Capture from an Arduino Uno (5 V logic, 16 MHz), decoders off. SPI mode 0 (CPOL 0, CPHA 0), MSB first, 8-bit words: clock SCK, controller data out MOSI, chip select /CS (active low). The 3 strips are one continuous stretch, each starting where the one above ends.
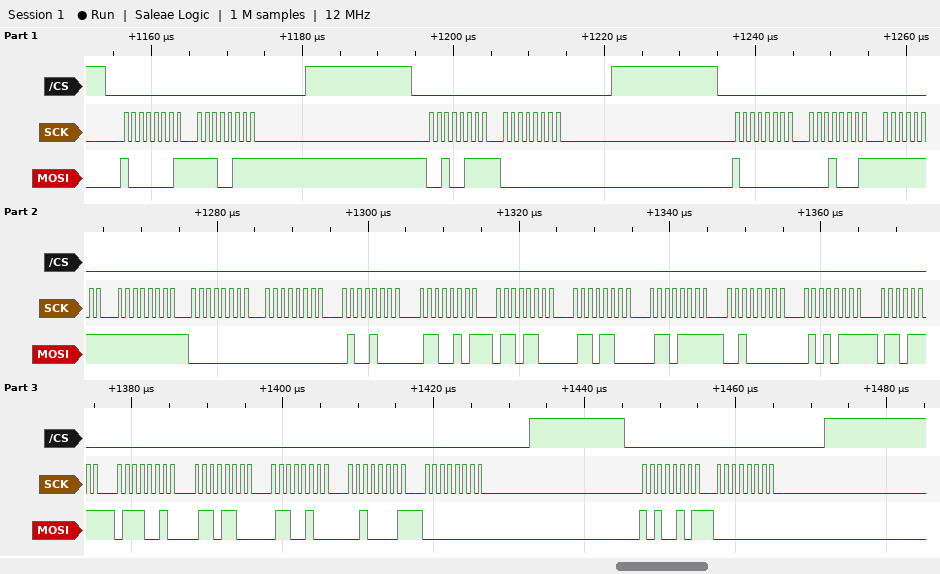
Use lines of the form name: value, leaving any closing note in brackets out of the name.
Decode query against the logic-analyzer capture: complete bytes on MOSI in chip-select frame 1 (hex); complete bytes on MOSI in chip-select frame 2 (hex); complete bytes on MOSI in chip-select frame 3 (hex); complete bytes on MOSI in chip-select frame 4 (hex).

complete bytes on MOSI in chip-select frame 1: 0x81 0xE7
complete bytes on MOSI in chip-select frame 2: 0x27 0x00
complete bytes on MOSI in chip-select frame 3: 0x80 0x11 0xFF 0xFF 0x00 0x00 0x48 0x65 0x6C 0x6C 0x6F 0x20 0x57 0x6F 0x72 0x6C 0x64 0x21 0x00
complete bytes on MOSI in chip-select frame 4: 0xA5 0x00
